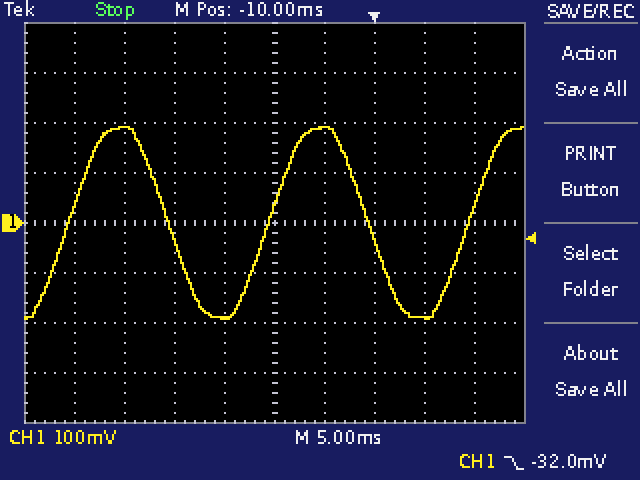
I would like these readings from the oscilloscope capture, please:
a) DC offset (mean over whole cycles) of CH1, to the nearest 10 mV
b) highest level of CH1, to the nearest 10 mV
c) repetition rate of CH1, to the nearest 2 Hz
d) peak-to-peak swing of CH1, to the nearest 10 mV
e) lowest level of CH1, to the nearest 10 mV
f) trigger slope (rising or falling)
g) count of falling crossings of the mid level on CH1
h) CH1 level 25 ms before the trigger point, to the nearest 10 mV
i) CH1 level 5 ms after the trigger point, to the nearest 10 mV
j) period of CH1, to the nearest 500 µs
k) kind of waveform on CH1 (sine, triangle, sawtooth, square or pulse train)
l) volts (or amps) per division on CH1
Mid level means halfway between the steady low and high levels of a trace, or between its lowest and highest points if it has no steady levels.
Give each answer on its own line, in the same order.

0 mV
190 mV
50 Hz
380 mV
-190 mV
falling
2
190 mV
-190 mV
20.0 ms
sine
100 mV
